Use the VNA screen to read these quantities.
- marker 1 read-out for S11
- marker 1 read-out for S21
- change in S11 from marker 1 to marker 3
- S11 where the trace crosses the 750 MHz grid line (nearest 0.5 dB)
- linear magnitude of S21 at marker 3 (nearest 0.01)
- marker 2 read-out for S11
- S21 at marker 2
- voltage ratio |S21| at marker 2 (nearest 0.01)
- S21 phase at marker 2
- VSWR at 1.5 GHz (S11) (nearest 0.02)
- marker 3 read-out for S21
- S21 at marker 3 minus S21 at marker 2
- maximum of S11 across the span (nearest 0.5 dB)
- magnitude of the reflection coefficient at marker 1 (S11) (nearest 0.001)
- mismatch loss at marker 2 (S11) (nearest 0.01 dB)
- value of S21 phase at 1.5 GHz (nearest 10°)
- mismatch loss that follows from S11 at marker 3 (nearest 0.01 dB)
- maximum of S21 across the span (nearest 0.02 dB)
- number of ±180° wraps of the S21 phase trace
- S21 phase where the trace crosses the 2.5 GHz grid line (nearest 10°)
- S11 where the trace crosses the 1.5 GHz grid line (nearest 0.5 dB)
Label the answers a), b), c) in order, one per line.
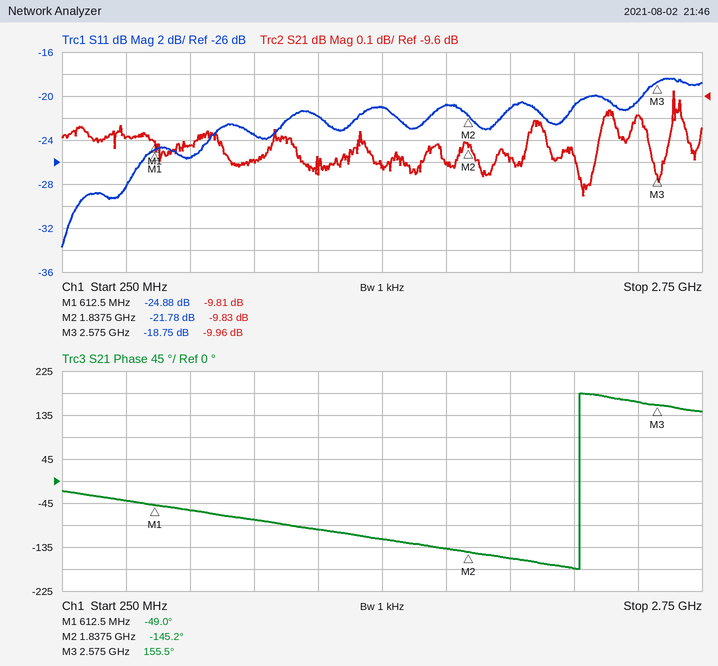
a) -24.88 dB
b) -9.81 dB
c) 6.13 dB
d) -25.5 dB
e) 0.32
f) -21.78 dB
g) -9.83 dB
h) 0.32
i) -145.2°
j) 1.20
k) -9.96 dB
l) -0.13 dB
m) -18.5 dB
n) 0.057
o) 0.03 dB
p) -120°
q) 0.06 dB
r) -9.58 dB
s) 1
t) 160°
u) -21.0 dB
